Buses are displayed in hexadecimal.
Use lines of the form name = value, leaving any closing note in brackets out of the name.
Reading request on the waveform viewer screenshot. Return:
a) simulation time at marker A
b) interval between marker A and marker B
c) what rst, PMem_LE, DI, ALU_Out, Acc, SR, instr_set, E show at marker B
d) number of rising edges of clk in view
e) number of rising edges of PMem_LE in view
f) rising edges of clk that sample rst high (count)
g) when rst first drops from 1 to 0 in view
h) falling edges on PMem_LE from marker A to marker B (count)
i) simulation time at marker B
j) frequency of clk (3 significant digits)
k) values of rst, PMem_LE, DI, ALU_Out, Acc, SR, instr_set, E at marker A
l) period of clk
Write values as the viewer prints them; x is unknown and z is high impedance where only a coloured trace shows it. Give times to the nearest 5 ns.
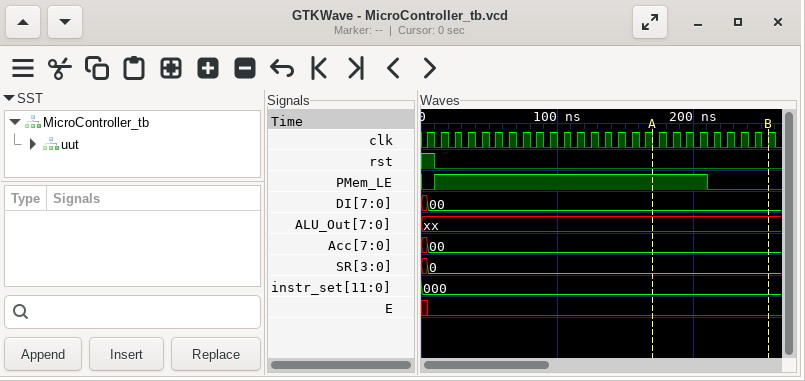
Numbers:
simulation time at marker A = 170 ns
interval between marker A and marker B = 85 ns
what rst, PMem_LE, DI, ALU_Out, Acc, SR, instr_set, E show at marker B = rst=0, PMem_LE=0, DI=00, ALU_Out=xx, Acc=00, SR=0, instr_set=000, E=0
number of rising edges of clk in view = 26
number of rising edges of PMem_LE in view = 1
rising edges of clk that sample rst high = 1
when rst first drops from 1 to 0 in view = 10 ns
falling edges on PMem_LE from marker A to marker B = 1
simulation time at marker B = 255 ns
frequency of clk = 100 MHz
values of rst, PMem_LE, DI, ALU_Out, Acc, SR, instr_set, E at marker A = rst=0, PMem_LE=1, DI=00, ALU_Out=xx, Acc=00, SR=0, instr_set=000, E=0
period of clk = 10 ns
